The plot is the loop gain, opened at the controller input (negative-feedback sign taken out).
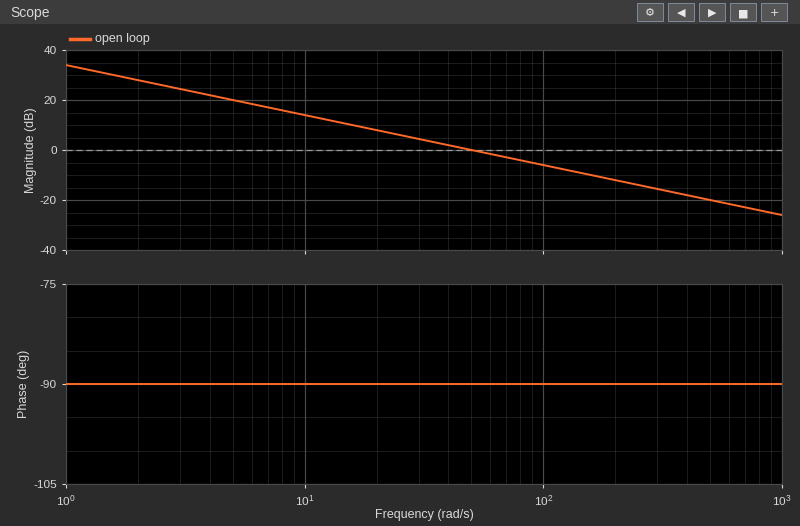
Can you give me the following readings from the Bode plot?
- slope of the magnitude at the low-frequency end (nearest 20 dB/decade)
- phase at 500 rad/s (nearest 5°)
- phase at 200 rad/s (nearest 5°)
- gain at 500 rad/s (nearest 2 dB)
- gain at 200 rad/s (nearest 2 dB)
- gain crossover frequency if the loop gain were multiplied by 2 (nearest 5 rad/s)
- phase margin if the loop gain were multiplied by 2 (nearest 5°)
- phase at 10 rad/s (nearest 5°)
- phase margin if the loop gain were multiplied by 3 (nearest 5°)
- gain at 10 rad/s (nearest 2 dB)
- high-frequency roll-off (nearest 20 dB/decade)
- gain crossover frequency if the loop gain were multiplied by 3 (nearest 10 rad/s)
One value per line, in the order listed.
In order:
-20 dB/decade
-90°
-90°
-20 dB
-12 dB
100 rad/s
90°
-90°
90°
14 dB
-20 dB/decade
150 rad/s
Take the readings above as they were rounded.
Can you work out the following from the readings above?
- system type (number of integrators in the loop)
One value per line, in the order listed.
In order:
1
